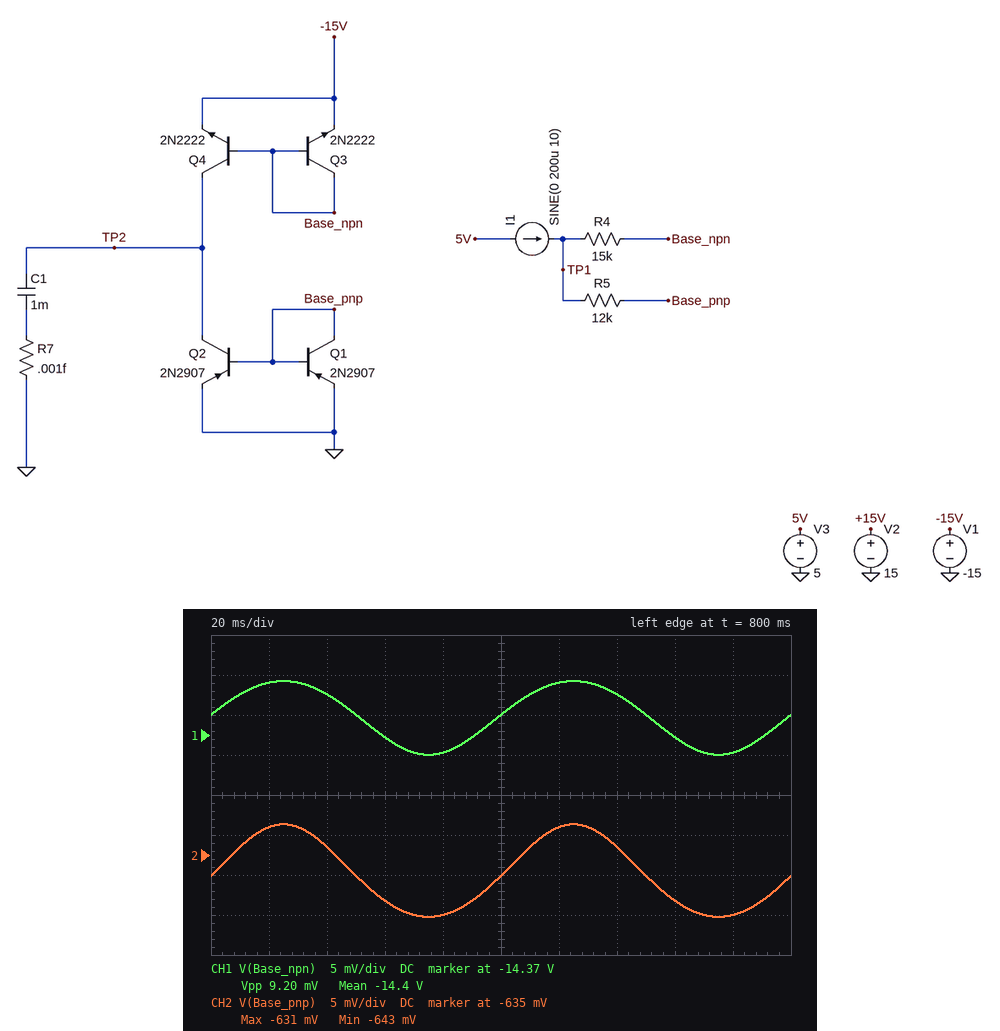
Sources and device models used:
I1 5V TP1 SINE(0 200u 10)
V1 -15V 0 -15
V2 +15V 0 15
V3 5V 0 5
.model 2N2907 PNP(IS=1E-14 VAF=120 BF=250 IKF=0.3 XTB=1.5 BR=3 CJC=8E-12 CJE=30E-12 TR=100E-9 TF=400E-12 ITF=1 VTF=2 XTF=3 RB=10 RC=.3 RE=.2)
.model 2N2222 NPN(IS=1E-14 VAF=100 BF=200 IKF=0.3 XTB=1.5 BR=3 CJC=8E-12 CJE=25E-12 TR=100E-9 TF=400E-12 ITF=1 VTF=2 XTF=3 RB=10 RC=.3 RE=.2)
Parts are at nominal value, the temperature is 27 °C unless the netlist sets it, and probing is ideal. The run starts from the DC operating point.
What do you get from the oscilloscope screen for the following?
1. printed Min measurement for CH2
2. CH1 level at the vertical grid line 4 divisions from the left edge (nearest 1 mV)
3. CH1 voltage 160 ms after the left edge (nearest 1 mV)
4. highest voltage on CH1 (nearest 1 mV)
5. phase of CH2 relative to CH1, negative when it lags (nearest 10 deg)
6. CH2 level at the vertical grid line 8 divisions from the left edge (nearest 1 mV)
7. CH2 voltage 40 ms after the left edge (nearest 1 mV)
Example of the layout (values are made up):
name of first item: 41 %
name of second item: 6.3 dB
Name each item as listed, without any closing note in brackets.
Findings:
printed Min measurement for CH2: -643 mV
CH1 level at the vertical grid line 4 divisions from the left edge: -14.367 V
CH1 voltage 160 ms after the left edge: -14.365 V
highest voltage on CH1: -14.358 V
phase of CH2 relative to CH1, negative when it lags: 0 deg
CH2 level at the vertical grid line 8 divisions from the left edge: -641 mV
CH2 voltage 40 ms after the left edge: -634 mV
